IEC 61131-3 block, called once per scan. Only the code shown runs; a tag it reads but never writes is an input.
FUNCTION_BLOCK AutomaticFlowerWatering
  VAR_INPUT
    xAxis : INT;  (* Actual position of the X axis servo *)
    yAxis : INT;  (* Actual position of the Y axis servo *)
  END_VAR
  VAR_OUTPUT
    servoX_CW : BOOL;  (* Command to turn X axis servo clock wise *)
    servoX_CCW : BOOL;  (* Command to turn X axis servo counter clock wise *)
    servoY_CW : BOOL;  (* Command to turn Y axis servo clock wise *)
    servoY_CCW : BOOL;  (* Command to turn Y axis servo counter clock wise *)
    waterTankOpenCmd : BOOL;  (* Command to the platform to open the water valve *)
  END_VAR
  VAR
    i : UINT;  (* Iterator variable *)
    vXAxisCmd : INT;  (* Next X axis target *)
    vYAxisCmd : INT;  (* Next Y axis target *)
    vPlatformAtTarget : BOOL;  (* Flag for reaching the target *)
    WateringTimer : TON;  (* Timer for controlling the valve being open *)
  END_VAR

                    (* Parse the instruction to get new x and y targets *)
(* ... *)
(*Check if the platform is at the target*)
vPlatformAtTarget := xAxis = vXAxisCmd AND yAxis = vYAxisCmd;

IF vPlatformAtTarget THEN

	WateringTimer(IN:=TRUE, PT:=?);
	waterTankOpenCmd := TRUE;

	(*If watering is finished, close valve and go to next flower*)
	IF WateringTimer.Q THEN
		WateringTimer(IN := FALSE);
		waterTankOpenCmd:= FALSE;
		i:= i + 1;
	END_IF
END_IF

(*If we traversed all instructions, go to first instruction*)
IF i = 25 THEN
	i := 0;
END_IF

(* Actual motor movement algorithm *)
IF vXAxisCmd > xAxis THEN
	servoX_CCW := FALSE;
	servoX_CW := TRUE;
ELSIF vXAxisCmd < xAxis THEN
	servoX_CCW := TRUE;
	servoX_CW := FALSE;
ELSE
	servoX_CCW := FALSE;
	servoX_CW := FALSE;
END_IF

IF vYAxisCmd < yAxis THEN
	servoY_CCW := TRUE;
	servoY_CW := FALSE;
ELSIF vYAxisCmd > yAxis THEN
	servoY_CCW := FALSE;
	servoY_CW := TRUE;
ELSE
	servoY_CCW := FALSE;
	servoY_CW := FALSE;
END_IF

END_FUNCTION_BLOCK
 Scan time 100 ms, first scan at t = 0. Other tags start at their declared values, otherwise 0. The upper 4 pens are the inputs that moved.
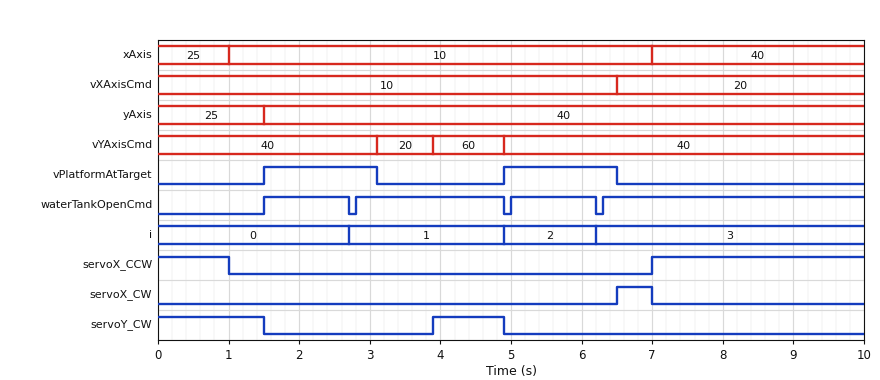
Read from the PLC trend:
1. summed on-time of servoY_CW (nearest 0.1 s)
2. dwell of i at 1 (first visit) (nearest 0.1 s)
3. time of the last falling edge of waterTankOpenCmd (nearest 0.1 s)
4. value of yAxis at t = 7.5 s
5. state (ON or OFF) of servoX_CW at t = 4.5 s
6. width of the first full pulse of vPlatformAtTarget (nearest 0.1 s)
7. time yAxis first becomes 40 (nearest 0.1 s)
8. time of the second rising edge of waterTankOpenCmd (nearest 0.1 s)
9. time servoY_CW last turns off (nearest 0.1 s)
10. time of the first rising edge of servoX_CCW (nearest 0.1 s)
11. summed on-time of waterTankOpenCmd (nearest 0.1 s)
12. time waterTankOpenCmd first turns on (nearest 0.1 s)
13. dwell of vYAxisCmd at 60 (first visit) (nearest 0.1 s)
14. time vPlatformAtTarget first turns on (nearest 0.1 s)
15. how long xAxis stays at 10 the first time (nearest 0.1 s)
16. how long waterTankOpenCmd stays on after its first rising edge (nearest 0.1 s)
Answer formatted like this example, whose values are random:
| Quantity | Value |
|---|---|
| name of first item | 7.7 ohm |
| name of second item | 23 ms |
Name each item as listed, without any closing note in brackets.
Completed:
| Quantity | Value |
|---|---|
| summed on-time of servoY_CW | 2.5 s |
| dwell of i at 1 (first visit) | 2.2 s |
| time of the last falling edge of waterTankOpenCmd | 6.2 s |
| value of yAxis at t = 7.5 s | 40 |
| state (ON or OFF) of servoX_CW at t = 4.5 s | OFF |
| width of the first full pulse of vPlatformAtTarget | 1.6 s |
| time yAxis first becomes 40 | 1.5 s |
| time of the second rising edge of waterTankOpenCmd | 2.8 s |
| time servoY_CW last turns off | 4.9 s |
| time of the first rising edge of servoX_CCW | 7.0 s |
| summed on-time of waterTankOpenCmd | 8.2 s |
| time waterTankOpenCmd first turns on | 1.5 s |
| dwell of vYAxisCmd at 60 (first visit) | 1.0 s |
| time vPlatformAtTarget first turns on | 1.5 s |
| how long xAxis stays at 10 the first time | 6.0 s |
| how long waterTankOpenCmd stays on after its first rising edge | 1.2 s |
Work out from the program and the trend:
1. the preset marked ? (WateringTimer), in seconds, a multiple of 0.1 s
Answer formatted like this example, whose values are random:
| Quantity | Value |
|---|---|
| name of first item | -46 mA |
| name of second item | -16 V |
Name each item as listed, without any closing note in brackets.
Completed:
| Quantity | Value |
|---|---|
| the preset marked ? (WateringTimer), in seconds, a multiple of 0.1 s | 1.2 s |
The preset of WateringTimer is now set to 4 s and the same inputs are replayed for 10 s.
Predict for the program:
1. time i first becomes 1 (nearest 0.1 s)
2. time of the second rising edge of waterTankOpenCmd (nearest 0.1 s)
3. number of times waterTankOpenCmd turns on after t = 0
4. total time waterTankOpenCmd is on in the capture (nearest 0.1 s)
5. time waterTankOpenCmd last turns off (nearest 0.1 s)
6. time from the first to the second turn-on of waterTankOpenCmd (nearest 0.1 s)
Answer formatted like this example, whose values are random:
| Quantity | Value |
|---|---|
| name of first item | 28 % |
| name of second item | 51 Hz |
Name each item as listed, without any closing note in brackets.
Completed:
| Quantity | Value |
|---|---|
| time i first becomes 1 | 5.5 s |
| time of the second rising edge of waterTankOpenCmd | 5.6 s |
| number of times waterTankOpenCmd turns on after t = 0 | 2 |
| total time waterTankOpenCmd is on in the capture | 8.4 s |
| time waterTankOpenCmd last turns off | 5.5 s |
| time from the first to the second turn-on of waterTankOpenCmd | 4.1 s |
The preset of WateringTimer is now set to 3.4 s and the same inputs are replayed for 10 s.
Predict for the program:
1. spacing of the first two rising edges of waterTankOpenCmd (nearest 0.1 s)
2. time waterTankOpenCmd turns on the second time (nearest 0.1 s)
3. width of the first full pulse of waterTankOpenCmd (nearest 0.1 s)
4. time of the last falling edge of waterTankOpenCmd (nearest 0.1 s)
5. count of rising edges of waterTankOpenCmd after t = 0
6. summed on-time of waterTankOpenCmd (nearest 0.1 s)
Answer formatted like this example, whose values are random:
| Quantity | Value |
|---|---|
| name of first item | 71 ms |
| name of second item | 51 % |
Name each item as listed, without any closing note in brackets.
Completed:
| Quantity | Value |
|---|---|
| spacing of the first two rising edges of waterTankOpenCmd | 3.5 s |
| time waterTankOpenCmd turns on the second time | 5.0 s |
| width of the first full pulse of waterTankOpenCmd | 3.4 s |
| time of the last falling edge of waterTankOpenCmd | 4.9 s |
| count of rising edges of waterTankOpenCmd after t = 0 | 2 |
| summed on-time of waterTankOpenCmd | 8.4 s |
